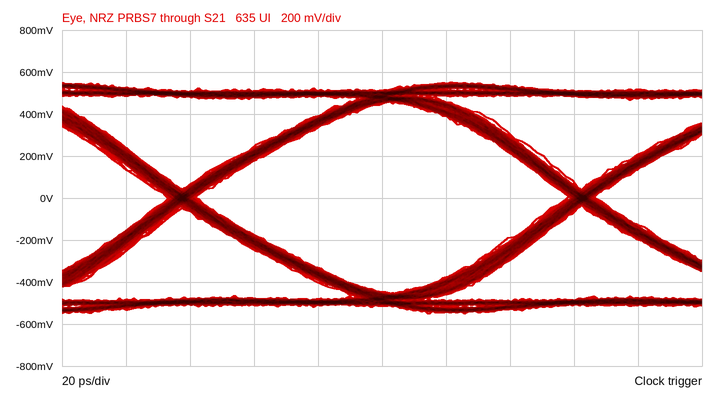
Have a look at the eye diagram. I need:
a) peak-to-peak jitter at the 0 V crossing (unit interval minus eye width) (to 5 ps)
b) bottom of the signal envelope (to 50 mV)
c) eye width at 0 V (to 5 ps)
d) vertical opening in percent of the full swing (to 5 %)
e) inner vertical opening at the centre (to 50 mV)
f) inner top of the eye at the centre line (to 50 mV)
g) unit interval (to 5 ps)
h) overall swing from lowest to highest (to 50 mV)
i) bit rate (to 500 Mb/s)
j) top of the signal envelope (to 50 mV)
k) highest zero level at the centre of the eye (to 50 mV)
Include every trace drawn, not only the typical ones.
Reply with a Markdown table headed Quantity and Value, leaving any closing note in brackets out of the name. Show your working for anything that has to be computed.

| Quantity | Value |
|---|---|
| peak-to-peak jitter at the 0 V crossing (unit interval minus eye width) | 10 ps |
| bottom of the signal envelope | -550 mV |
| eye width at 0 V | 115 ps |
| vertical opening in percent of the full swing | 900 mV / 1.10 V ≈ 81.8 %, so 80 % to the nearest 5 % |
| inner vertical opening at the centre | 900 mV |
| inner top of the eye at the centre line | 450 mV |
| unit interval | 125 ps |
| overall swing from lowest to highest | 1.10 V |
| bit rate | 8.0 Gb/s |
| top of the signal envelope | 550 mV |
| highest zero level at the centre of the eye | -450 mV |
